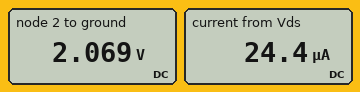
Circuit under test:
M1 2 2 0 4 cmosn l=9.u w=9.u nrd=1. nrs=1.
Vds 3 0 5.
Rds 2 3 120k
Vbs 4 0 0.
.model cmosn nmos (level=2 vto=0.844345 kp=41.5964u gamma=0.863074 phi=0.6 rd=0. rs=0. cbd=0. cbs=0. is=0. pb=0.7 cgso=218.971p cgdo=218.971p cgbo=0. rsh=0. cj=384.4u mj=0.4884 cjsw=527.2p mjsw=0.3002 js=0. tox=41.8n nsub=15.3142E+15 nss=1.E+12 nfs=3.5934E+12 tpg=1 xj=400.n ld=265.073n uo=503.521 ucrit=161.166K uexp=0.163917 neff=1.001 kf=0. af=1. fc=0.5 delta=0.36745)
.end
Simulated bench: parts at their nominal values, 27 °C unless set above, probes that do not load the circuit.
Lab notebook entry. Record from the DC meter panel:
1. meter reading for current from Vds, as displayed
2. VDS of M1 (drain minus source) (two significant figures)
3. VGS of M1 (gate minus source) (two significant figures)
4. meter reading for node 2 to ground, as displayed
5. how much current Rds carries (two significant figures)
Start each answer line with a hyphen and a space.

- 24.4 µA
- 2.1 V
- 2.1 V
- 2.069 V
- 24 µA
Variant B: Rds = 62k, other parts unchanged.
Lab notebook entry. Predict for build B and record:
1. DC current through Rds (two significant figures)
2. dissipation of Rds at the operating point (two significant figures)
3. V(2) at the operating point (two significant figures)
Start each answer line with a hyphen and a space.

- 41 µA
- 110 µW
- 2.4 V
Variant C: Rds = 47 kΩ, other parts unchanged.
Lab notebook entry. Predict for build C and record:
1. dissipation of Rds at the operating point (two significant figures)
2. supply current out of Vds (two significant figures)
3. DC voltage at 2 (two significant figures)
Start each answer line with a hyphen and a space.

- 120 µW
- 51 µA
- 2.6 V
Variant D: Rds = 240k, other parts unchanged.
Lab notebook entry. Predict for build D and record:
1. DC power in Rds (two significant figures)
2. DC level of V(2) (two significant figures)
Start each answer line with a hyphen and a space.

- 44 µW
- 1.8 V
